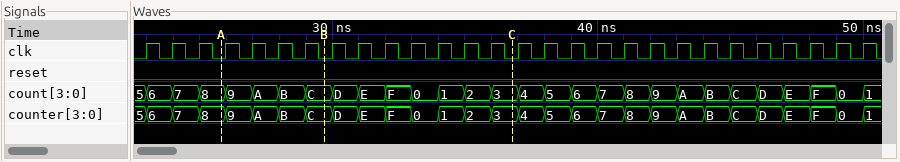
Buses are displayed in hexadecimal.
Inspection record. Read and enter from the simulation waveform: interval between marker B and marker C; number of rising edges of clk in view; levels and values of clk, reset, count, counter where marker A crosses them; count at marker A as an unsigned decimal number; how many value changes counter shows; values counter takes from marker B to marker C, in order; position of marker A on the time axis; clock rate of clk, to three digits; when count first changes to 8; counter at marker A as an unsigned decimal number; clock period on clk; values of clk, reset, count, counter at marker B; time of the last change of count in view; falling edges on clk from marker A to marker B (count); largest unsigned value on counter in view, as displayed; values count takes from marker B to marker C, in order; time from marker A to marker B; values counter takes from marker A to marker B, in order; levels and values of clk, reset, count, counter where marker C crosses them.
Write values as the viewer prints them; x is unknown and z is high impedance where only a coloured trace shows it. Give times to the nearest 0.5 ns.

7 ns
28
clk=0, reset=0, count=8, counter=8
8
28
C, D, E, F, 0, 1, 2, 3
26 ns
1.00 GHz
25 ns
8
1 ns
clk=0, reset=0, count=C, counter=C
50 ns
4
F
C, D, E, F, 0, 1, 2, 3
4 ns
8, 9, A, B, C
clk=0, reset=0, count=3, counter=3
